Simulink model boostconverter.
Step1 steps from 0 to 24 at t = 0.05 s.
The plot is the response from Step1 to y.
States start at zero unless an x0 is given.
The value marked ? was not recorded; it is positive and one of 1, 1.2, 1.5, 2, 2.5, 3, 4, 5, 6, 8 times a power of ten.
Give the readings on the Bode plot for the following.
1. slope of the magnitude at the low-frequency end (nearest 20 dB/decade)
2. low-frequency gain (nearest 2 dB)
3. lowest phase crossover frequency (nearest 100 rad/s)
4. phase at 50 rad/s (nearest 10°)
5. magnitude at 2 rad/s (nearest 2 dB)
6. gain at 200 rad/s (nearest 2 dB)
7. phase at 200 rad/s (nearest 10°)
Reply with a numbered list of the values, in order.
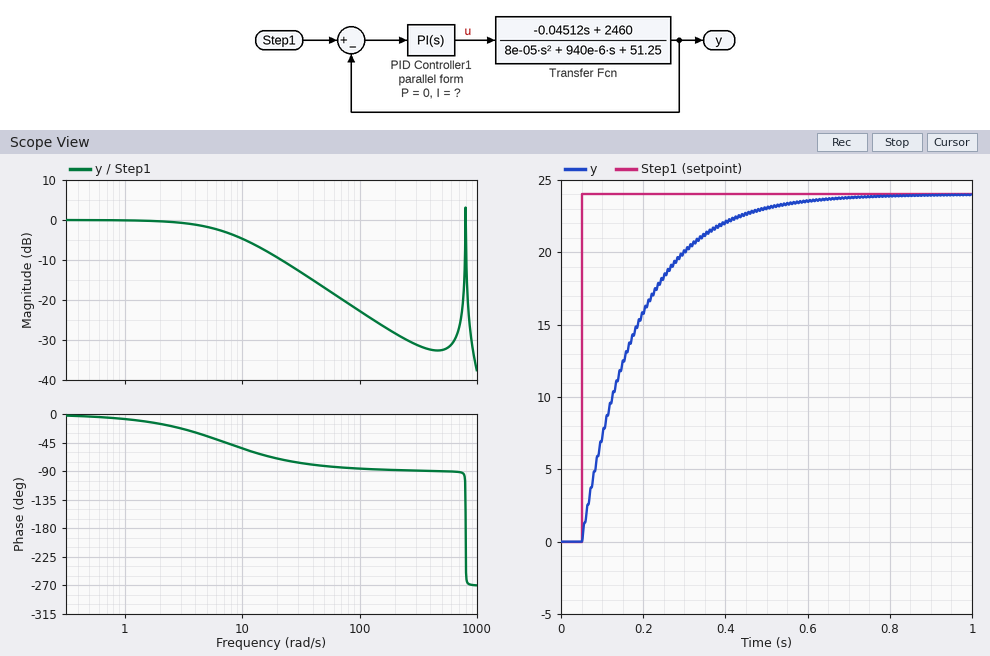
1. 0 dB/decade
2. 0 dB
3. 800 rad/s
4. -80°
5. 0 dB
6. -28 dB
7. -90°
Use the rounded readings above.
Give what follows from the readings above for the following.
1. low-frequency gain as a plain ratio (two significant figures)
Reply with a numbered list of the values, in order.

1. 1.0
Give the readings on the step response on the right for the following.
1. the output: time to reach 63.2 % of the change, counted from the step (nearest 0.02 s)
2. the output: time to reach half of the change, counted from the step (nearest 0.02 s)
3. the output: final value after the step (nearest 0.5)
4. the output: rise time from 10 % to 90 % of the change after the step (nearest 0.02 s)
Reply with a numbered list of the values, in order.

1. 0.14 s
2. 0.10 s
3. 24.0
4. 0.30 s
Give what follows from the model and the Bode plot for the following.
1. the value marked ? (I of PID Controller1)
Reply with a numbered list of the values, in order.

1. 0.15
